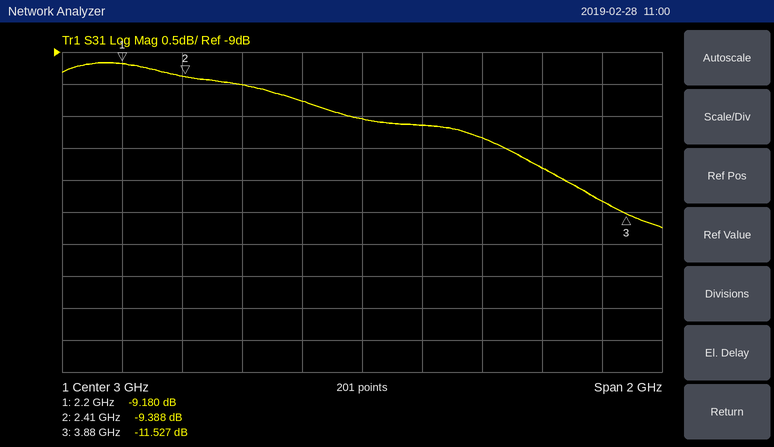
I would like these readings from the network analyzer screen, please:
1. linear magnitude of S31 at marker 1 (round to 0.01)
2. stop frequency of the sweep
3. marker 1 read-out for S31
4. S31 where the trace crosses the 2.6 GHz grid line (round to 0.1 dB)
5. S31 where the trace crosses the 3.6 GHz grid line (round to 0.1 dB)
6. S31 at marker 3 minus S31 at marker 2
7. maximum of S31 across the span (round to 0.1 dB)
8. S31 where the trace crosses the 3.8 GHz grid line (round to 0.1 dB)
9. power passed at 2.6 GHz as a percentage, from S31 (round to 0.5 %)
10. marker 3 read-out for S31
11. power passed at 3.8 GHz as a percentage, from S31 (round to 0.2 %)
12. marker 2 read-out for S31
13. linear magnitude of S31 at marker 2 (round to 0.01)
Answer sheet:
0.35
4 GHz
-9.180 dB
-9.5 dB
-10.8 dB
-2.139 dB
-9.2 dB
-11.3 dB
11.0 %
-11.527 dB
7.4 %
-9.388 dB
0.34
